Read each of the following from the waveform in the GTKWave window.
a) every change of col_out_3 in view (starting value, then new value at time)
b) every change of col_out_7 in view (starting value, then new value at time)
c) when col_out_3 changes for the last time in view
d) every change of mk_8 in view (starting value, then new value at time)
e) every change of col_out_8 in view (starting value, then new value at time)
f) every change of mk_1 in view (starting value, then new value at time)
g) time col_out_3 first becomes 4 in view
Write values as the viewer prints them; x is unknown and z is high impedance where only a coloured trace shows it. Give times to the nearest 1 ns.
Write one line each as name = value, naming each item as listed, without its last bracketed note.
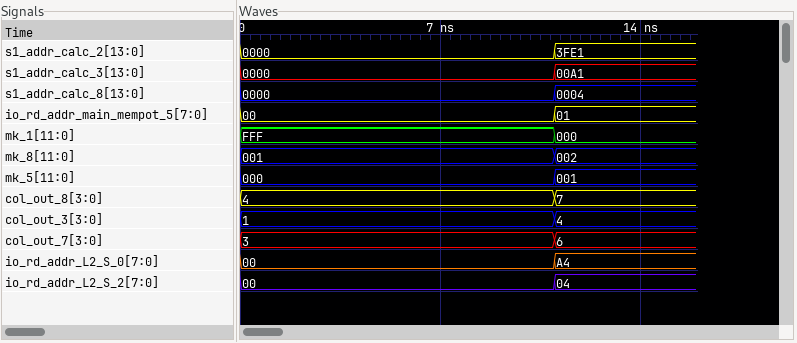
every change of col_out_3 in view = 1, 4 at 11 ns
every change of col_out_7 in view = 3, 6 at 11 ns
when col_out_3 changes for the last time in view = 11 ns
every change of mk_8 in view = 001, 002 at 11 ns
every change of col_out_8 in view = 4, 7 at 11 ns
every change of mk_1 in view = FFF, 000 at 11 ns
time col_out_3 first becomes 4 in view = 11 ns
